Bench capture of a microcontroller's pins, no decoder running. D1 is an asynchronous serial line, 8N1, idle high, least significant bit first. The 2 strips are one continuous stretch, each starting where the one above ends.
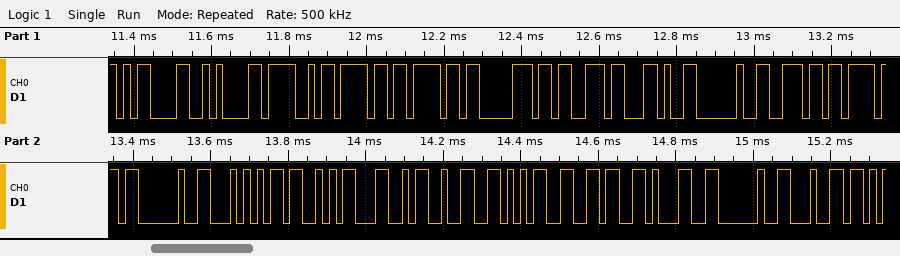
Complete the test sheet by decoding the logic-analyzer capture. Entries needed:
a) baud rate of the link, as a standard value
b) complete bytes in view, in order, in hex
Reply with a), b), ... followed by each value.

a) 57600 baud
b) 0D 0A 4F 6F 6F 70 73 2C 20 6E 6F 20 54 53 4C 32 35 36 31 20 64
